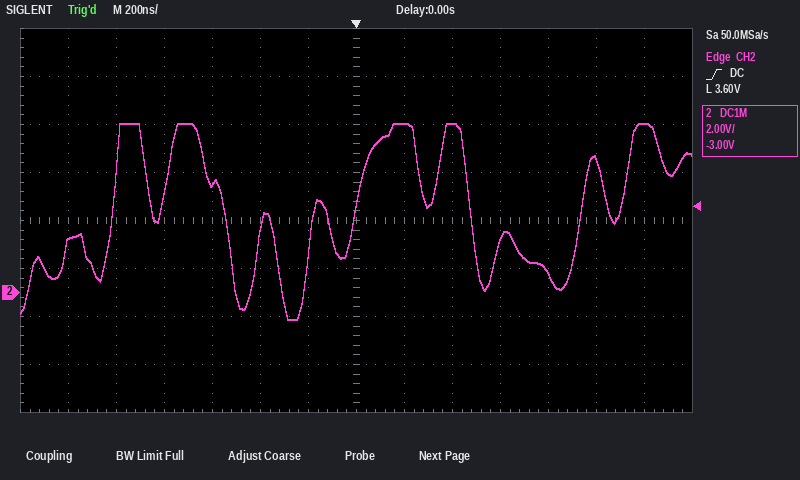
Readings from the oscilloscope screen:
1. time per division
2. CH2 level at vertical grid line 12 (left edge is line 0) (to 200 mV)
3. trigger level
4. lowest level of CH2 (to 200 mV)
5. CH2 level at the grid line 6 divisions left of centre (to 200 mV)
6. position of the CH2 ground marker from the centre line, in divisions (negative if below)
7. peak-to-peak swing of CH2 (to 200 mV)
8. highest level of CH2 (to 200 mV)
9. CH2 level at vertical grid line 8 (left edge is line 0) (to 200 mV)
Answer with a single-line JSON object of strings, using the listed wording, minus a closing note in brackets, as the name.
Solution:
{"time per division": "200 ns", "CH2 level at vertical grid line 12 (left edge is line 0)": "5.6 V", "trigger level": "3.60 V", "lowest level of CH2": "-1.2 V", "CH2 level at the grid line 6 divisions left of centre": "2.2 V", "position of the CH2 ground marker from the centre line, in divisions": "-1.5 div", "peak-to-peak swing of CH2": "8.2 V", "highest level of CH2": "7.0 V", "CH2 level at vertical grid line 8 (left edge is line 0)": "7.0 V"}
